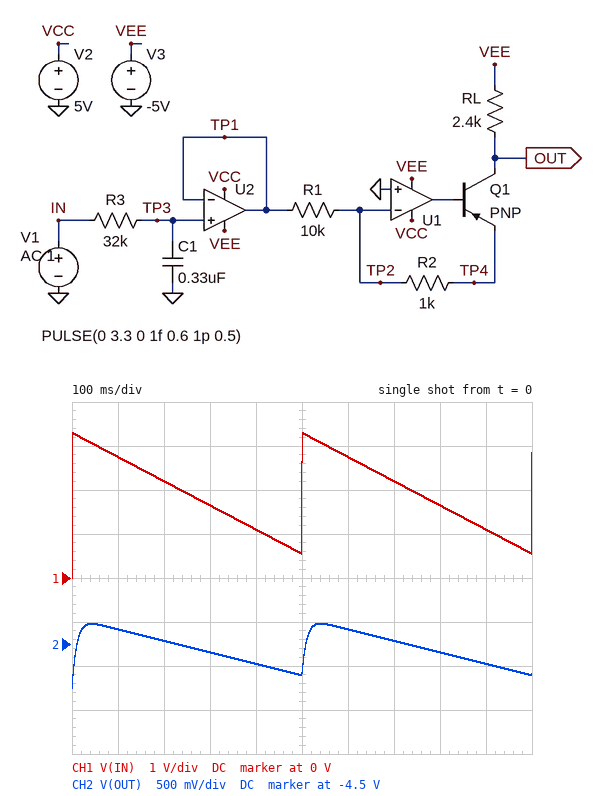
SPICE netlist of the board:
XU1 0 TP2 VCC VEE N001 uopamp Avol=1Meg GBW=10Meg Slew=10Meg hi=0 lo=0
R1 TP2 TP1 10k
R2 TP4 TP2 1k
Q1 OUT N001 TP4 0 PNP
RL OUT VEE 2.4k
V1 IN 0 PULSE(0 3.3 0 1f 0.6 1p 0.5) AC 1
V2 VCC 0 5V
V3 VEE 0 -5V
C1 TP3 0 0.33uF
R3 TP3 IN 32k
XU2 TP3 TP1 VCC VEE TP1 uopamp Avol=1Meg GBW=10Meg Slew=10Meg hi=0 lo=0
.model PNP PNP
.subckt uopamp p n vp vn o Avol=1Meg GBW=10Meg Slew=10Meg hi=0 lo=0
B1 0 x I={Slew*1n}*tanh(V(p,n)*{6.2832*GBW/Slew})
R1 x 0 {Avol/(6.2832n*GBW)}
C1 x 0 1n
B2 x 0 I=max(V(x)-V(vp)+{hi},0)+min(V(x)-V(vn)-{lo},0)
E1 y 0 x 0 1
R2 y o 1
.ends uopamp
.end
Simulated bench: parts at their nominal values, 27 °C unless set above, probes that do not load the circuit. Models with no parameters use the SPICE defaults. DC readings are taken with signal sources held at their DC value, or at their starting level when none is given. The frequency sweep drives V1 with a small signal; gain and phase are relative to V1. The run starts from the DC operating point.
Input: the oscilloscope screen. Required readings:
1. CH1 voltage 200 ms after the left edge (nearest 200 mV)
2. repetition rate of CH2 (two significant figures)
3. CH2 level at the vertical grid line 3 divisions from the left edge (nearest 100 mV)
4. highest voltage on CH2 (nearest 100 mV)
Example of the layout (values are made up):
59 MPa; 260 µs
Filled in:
2.2 V; 2.0 Hz; -4.6 V; -4.3 V
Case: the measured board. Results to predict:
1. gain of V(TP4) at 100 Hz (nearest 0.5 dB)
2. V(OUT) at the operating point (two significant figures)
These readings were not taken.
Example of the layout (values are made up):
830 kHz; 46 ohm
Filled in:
-16.5 dB; -5.0 V
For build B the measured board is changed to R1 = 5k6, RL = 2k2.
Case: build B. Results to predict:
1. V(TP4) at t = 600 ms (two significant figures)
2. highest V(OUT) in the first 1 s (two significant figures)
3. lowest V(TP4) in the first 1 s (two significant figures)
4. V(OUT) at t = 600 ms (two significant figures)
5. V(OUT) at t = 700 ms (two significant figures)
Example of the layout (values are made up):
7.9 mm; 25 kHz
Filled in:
-500 mV; -3.8 V; -550 mV; -3.9 V; -4.1 V
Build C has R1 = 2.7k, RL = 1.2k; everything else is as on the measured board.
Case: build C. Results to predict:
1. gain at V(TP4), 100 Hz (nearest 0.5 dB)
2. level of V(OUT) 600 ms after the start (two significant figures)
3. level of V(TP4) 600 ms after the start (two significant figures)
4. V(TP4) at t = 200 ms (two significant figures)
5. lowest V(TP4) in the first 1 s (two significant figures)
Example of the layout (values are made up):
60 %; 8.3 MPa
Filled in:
-16.5 dB; -3.8 V; -1.0 V; -840 mV; -1.1 V
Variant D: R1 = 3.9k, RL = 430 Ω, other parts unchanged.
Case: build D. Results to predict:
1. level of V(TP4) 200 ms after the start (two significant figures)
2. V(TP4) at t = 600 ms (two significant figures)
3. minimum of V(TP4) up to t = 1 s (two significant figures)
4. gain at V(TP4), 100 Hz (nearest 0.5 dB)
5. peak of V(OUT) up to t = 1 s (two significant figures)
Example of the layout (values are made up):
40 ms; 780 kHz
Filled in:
-580 mV; -720 mV; -790 mV; -16.5 dB; -4.7 V
